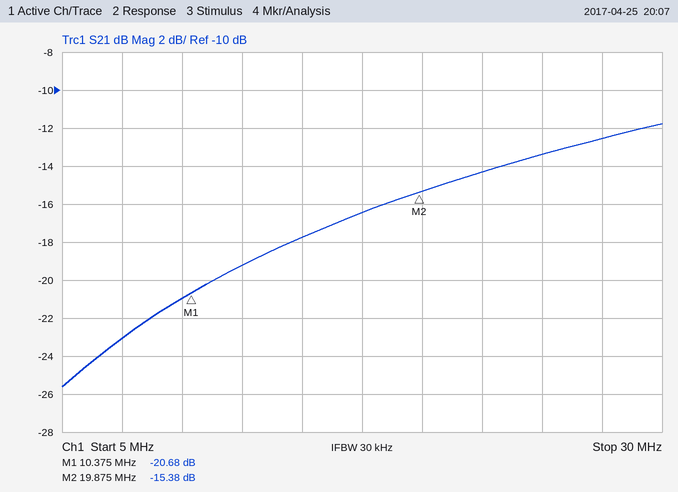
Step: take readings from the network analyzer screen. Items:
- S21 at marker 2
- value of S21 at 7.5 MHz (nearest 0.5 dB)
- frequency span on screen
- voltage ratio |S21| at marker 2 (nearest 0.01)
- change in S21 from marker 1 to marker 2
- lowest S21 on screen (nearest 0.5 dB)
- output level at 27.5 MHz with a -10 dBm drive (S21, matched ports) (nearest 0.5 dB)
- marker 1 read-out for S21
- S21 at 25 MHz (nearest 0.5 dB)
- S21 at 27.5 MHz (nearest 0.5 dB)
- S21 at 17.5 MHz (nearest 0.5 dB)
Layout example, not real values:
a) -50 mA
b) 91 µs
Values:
a) -15.38 dB
b) -23.0 dB
c) 25 MHz
d) 0.17
e) 5.30 dB
f) -25.5 dB
g) -22.5 dBm
h) -20.68 dB
i) -13.5 dB
j) -12.5 dB
k) -16.5 dB
